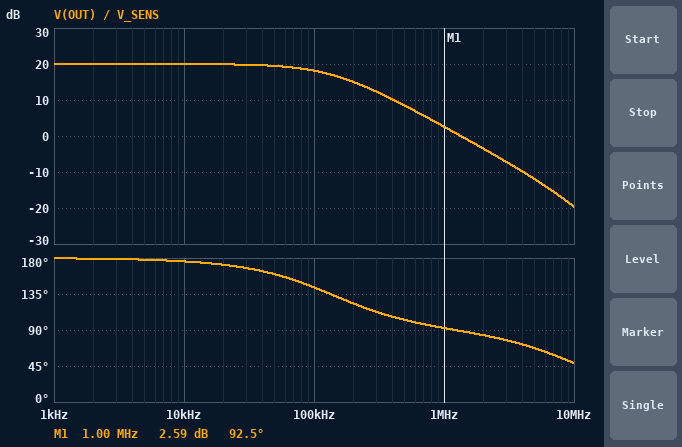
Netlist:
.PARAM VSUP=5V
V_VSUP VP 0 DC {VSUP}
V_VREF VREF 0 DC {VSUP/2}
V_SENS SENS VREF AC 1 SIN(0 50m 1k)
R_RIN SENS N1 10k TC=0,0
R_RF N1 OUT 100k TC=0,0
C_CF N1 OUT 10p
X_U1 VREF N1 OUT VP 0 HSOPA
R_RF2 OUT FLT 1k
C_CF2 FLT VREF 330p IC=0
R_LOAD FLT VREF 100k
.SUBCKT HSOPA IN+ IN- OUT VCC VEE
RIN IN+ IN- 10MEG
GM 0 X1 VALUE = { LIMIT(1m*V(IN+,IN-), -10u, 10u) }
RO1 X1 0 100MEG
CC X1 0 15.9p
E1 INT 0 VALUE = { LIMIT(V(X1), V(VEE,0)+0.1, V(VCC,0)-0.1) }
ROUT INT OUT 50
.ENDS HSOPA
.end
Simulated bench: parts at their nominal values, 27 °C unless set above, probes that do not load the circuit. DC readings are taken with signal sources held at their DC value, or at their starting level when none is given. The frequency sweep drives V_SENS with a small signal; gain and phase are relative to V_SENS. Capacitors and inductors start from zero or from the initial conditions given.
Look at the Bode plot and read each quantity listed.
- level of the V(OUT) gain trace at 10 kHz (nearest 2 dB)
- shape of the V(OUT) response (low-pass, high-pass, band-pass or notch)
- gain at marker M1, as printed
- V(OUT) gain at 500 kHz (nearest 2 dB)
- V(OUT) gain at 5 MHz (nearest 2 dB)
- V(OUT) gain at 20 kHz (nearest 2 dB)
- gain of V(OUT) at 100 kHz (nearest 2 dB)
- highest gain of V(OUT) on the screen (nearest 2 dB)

20 dB
low-pass
2.59 dB
8 dB
-12 dB
20 dB
18 dB
20 dB
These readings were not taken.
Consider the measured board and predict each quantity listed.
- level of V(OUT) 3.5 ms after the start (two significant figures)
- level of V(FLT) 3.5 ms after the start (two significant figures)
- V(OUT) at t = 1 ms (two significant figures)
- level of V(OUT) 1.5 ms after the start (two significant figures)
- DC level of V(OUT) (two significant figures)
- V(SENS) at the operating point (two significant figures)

2.5 V
2.5 V
2.5 V
2.5 V
2.5 V
2.5 V
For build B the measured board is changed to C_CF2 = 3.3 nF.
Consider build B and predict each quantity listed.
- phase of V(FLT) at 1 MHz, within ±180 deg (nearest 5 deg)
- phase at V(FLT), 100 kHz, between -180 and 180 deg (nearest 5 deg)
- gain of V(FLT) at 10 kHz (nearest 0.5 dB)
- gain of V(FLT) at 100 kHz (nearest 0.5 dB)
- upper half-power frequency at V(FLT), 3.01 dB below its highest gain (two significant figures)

5 deg
80 deg
19.5 dB
11.0 dB
44 kHz
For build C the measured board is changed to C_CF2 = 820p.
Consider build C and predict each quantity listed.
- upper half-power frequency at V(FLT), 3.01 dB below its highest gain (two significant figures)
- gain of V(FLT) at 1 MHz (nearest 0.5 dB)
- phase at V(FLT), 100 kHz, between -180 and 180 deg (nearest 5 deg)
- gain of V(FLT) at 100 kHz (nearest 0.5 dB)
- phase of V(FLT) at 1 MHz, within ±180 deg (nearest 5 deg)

100 kHz
-12.0 dB
115 deg
17.0 dB
15 deg
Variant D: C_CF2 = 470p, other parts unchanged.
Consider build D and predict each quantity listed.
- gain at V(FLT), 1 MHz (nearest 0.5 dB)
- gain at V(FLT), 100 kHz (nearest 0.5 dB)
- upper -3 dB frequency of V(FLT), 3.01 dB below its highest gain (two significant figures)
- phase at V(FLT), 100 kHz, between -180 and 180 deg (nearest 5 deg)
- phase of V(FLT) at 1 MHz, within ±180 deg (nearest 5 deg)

-7.5 dB
17.5 dB
120 kHz
125 deg
20 deg
